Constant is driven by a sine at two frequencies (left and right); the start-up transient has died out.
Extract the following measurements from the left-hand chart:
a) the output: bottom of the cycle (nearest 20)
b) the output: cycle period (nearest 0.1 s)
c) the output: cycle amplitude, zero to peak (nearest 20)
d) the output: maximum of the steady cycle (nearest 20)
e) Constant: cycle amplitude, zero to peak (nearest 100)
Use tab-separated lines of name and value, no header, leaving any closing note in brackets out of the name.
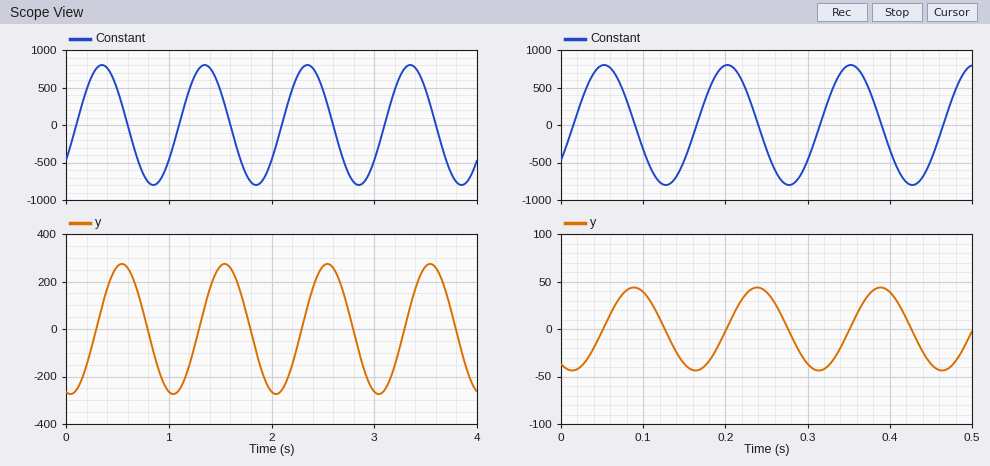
the output: bottom of the cycle	-280
the output: cycle period	1.0 s
the output: cycle amplitude, zero to peak	280
the output: maximum of the steady cycle	280
Constant: cycle amplitude, zero to peak	800
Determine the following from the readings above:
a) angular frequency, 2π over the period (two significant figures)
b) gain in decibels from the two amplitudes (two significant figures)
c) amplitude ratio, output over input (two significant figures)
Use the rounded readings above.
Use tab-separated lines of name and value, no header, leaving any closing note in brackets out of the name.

angular frequency, 2π over the period	6.3 rad/s
gain in decibels from the two amplitudes	-9.1 dB
amplitude ratio, output over input	0.35
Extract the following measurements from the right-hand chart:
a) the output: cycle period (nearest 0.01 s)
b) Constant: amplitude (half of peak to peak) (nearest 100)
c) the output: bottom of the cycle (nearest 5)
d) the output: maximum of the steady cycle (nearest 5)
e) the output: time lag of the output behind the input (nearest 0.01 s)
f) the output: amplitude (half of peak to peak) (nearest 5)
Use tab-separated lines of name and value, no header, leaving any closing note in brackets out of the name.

the output: cycle period	0.15 s
Constant: amplitude (half of peak to peak)	800
the output: bottom of the cycle	-45
the output: maximum of the steady cycle	45
the output: time lag of the output behind the input	0.04 s
the output: amplitude (half of peak to peak)	45
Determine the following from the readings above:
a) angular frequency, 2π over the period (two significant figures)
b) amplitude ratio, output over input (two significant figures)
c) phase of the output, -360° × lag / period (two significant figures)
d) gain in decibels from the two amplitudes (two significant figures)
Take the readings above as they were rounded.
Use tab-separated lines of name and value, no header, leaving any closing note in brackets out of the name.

angular frequency, 2π over the period	42 rad/s
amplitude ratio, output over input	0.056
phase of the output, -360° × lag / period	-96°
gain in decibels from the two amplitudes	-25 dB
